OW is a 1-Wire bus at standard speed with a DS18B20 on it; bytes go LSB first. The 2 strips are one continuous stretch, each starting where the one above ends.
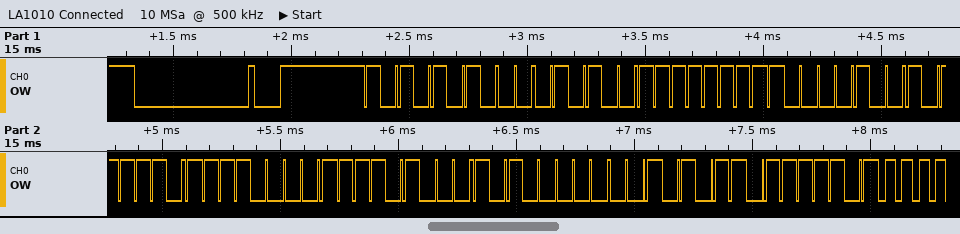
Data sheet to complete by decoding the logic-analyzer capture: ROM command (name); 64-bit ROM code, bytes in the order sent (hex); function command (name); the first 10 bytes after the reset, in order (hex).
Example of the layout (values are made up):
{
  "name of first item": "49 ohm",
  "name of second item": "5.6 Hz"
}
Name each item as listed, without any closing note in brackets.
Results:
{
  "ROM command": "Match ROM",
  "64-bit ROM code, bytes in the order sent": "28 FF 21 BD 87 17 05 D4",
  "function command": "Read Scratchpad",
  "the first 10 bytes after the reset, in order": "55 28 FF 21 BD 87 17 05 D4 BE"
}
